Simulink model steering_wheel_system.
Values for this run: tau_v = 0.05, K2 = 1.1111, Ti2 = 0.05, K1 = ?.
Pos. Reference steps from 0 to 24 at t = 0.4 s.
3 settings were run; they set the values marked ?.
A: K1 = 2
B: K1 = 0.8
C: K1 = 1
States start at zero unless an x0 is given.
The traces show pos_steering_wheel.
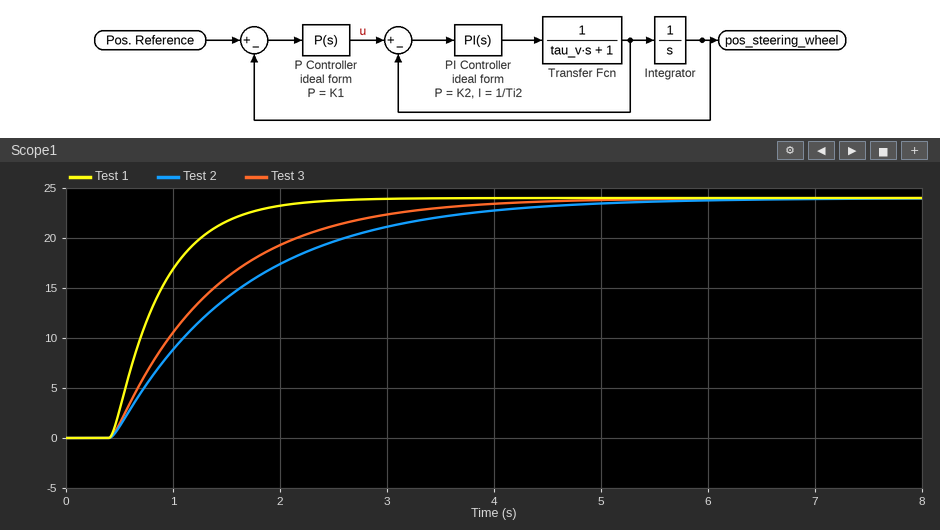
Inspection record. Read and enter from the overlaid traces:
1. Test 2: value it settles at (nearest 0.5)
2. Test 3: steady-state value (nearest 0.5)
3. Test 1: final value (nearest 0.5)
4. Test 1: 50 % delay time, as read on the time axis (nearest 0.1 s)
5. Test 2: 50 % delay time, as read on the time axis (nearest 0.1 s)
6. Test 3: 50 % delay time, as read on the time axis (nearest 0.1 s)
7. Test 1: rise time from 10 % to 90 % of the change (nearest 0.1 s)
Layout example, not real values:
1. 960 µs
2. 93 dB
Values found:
1. 24.0
2. 24.0
3. 24.0
4. 0.8 s
5. 1.3 s
6. 1.1 s
7. 1.0 s
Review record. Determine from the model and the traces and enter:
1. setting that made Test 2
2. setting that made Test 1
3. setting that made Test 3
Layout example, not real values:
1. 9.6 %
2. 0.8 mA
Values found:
1. B
2. A
3. C
